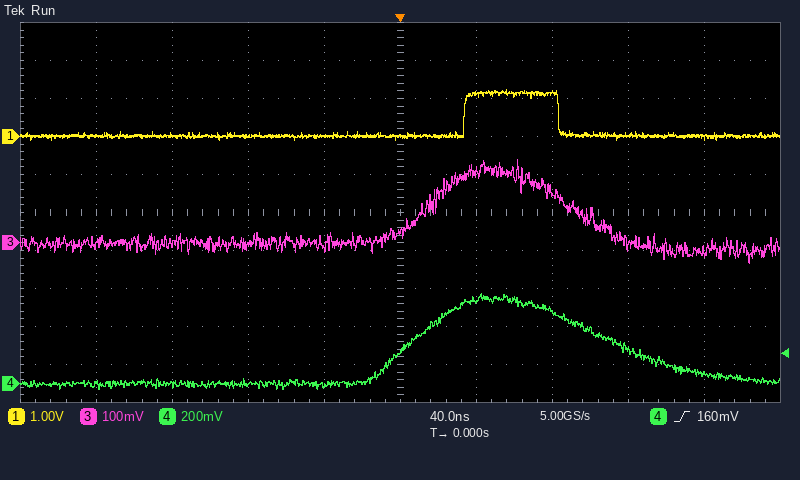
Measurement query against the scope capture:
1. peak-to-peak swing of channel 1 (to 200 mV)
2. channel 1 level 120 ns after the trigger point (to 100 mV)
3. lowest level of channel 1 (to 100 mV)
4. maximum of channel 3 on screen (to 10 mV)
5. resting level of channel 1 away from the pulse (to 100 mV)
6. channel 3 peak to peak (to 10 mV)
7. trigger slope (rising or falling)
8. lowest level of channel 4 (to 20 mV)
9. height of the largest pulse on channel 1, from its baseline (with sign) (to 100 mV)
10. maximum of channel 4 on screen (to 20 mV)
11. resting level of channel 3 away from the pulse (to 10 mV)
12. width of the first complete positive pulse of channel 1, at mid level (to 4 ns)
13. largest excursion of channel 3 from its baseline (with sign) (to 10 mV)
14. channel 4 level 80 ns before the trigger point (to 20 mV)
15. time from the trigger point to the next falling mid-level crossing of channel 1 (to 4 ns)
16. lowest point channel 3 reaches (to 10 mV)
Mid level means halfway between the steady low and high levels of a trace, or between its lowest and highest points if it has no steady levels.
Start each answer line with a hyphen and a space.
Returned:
- 1.4 V
- 0.0 V
- -100 mV
- 220 mV
- 0.0 V
- 270 mV
- rising
- -40 mV
- +1.2 V
- 480 mV
- 0 mV
- 48 ns
- +220 mV
- 0 mV
- 84 ns
- -50 mV
